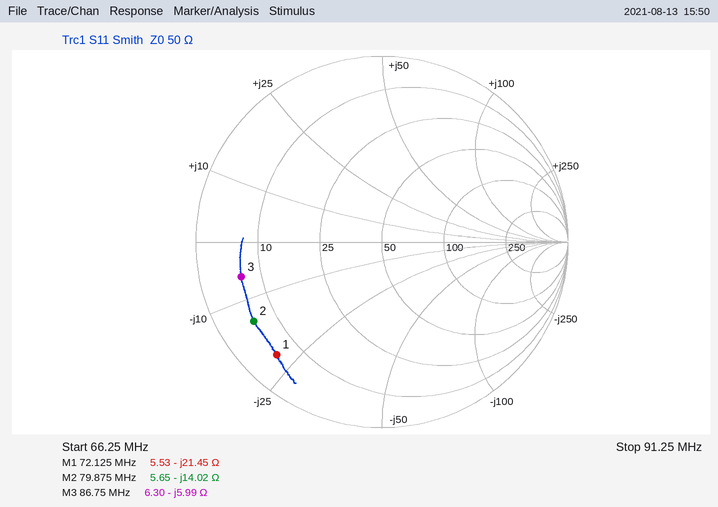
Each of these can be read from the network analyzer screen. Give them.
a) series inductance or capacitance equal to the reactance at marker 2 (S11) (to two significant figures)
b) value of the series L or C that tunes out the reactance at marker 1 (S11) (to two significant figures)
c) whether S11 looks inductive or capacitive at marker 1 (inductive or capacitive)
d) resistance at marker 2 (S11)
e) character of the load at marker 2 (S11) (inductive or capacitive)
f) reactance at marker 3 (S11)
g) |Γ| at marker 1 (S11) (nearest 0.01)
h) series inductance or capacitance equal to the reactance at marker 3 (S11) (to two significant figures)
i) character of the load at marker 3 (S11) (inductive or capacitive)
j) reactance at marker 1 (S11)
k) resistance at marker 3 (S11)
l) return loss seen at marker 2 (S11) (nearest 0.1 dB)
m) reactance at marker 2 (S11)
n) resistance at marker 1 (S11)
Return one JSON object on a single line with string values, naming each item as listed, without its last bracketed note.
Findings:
{"series inductance or capacitance equal to the reactance at marker 2 (S11)": "140 pF", "value of the series L or C that tunes out the reactance at marker 1 (S11)": "47 nH", "whether S11 looks inductive or capacitive at marker 1": "capacitive", "resistance at marker 2": "5.65 Ω", "character of the load at marker 2 (S11)": "capacitive", "reactance at marker 3": "-5.99 Ω", "|Γ| at marker 1 (S11)": "0.83", "series inductance or capacitance equal to the reactance at marker 3 (S11)": "310 pF", "character of the load at marker 3 (S11)": "capacitive", "reactance at marker 1": "-21.45 Ω", "resistance at marker 3": "6.30 Ω", "return loss seen at marker 2 (S11)": "1.8 dB", "reactance at marker 2": "-14.02 Ω", "resistance at marker 1": "5.53 Ω"}
